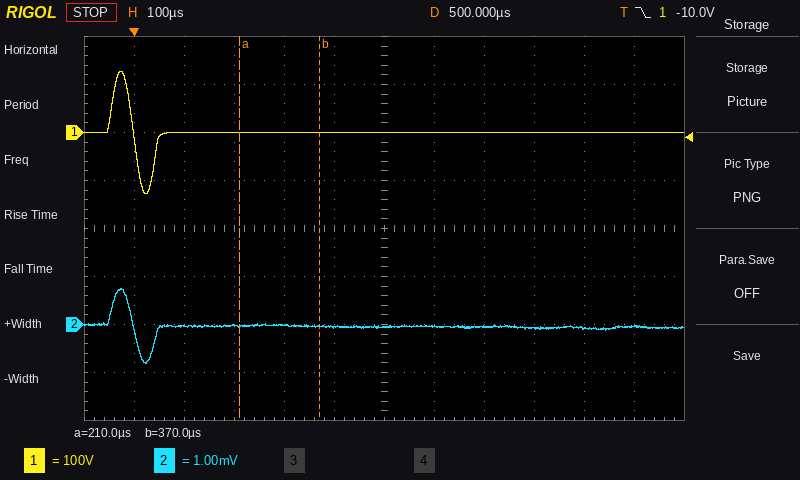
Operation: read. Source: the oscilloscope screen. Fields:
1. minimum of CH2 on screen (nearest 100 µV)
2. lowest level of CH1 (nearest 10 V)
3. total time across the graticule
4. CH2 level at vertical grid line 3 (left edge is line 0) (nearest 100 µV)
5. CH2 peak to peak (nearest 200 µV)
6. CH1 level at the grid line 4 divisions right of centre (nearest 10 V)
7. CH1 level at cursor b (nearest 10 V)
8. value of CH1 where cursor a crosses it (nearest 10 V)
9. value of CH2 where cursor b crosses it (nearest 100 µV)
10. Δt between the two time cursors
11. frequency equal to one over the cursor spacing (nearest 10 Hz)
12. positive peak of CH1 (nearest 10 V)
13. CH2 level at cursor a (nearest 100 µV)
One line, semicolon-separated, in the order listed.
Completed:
-800 µV; -130 V; 1.2 ms; 0.0 mV; 1.6 mV; 0 V; 0 V; 0 V; 0.0 mV; 160 µs; 6.25 kHz; 130 V; 0.0 mV
